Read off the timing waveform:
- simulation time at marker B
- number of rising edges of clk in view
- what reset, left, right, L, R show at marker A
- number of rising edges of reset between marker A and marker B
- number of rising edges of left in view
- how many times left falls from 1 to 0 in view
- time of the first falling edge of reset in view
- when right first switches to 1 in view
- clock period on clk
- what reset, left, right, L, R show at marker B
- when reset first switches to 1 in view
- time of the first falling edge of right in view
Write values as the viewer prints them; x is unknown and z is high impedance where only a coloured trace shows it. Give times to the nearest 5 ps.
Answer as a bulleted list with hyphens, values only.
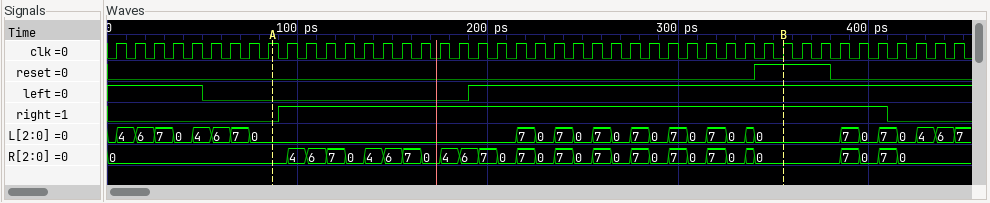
- 355 ps
- 45
- reset=0, left=0, right=0, L=0, R=0
- 1
- 1
- 1
- 380 ps
- 90 ps
- 10 ps
- reset=1, left=1, right=1, L=0, R=0
- 340 ps
- 410 ps
